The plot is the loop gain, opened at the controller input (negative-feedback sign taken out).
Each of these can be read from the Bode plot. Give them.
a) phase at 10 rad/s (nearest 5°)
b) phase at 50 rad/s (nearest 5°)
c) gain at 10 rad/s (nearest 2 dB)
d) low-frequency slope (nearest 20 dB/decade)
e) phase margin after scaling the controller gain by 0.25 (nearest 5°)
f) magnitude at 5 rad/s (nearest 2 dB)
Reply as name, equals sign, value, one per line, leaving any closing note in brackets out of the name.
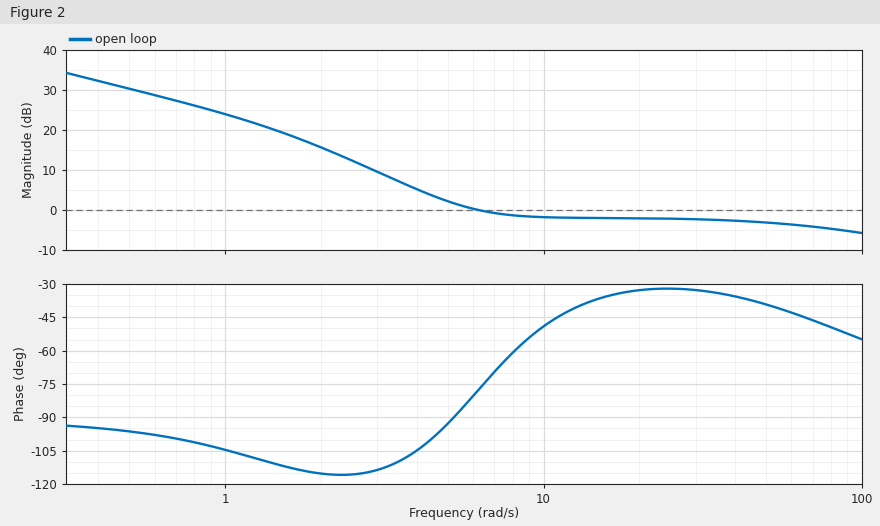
phase at 10 rad/s = -50°
phase at 50 rad/s = -40°
gain at 10 rad/s = -2 dB
low-frequency slope = -20 dB/decade
phase margin after scaling the controller gain by 0.25 = 65°
magnitude at 5 rad/s = 2 dB
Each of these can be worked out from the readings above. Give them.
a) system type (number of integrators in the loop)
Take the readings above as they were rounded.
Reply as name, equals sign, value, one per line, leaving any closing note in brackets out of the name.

system type = 1
